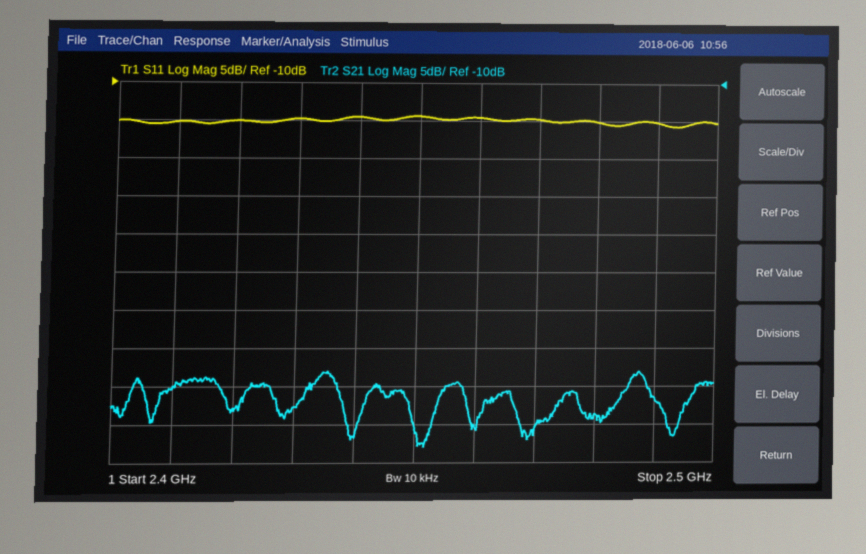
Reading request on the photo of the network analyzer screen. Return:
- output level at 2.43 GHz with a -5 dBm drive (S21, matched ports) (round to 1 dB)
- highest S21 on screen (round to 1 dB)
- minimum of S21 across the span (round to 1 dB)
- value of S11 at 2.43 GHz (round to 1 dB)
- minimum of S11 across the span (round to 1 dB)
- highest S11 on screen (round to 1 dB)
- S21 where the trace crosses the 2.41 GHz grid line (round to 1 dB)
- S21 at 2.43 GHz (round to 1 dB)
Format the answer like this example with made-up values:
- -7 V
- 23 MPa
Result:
- -58 dBm
- -48 dB
- -58 dB
- -15 dB
- -16 dB
- -14 dB
- -50 dB
- -53 dB
